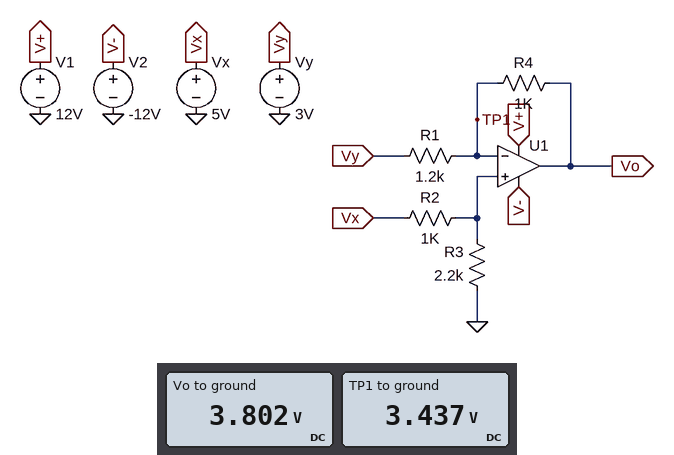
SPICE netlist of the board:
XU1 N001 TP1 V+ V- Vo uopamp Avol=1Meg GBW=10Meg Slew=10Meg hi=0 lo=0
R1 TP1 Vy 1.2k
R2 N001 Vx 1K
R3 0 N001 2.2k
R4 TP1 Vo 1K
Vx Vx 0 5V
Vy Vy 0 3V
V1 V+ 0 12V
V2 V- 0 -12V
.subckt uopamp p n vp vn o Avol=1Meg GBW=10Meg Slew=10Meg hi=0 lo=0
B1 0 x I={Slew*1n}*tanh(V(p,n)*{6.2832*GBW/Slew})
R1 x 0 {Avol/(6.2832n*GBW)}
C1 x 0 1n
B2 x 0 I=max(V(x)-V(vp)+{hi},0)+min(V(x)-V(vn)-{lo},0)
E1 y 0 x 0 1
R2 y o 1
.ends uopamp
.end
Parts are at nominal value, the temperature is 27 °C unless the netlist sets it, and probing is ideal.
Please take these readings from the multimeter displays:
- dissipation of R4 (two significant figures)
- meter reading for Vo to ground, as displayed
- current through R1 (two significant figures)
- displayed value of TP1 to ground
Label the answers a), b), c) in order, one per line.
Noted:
a) 130 µW
b) 3.802 V
c) 360 µA
d) 3.437 V
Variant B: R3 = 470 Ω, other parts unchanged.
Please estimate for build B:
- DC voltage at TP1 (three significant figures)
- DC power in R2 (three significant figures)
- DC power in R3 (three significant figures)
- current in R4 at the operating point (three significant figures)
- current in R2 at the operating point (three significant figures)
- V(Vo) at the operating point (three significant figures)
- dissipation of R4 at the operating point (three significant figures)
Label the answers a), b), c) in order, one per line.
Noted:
a) 1.60 V
b) 11.6 mW
c) 5.44 mW
d) 1.17 mA
e) 3.40 mA
f) 431 mV
g) 1.36 mW
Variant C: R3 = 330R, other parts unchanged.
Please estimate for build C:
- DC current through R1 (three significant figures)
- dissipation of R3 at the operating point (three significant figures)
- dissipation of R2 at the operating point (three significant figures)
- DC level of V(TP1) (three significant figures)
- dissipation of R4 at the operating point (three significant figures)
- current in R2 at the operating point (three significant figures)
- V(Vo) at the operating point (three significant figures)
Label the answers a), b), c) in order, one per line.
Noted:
a) 1.47 mA
b) 4.66 mW
c) 14.1 mW
d) 1.24 V
e) 2.15 mW
f) 3.76 mA
g) -226 mV
